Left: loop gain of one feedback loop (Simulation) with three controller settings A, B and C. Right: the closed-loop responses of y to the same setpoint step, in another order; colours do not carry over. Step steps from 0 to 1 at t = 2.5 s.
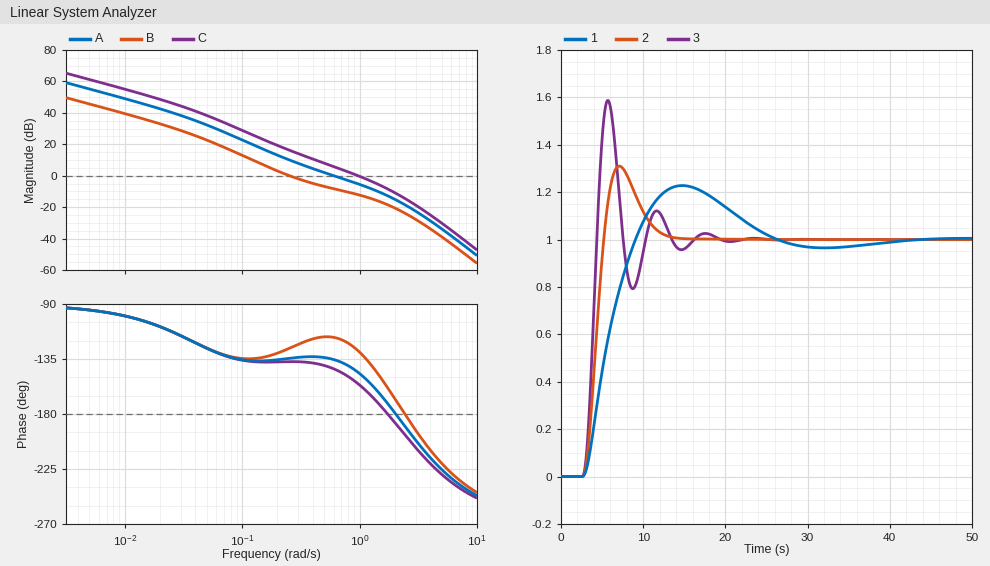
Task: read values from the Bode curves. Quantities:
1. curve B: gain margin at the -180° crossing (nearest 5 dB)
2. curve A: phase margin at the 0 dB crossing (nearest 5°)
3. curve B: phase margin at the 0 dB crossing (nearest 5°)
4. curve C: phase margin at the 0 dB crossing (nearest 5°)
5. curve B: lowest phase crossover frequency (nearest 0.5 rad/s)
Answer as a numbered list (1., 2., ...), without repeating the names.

1. 25 dB
2. 45°
3. 55°
4. 25°
5. 2.5 rad/s
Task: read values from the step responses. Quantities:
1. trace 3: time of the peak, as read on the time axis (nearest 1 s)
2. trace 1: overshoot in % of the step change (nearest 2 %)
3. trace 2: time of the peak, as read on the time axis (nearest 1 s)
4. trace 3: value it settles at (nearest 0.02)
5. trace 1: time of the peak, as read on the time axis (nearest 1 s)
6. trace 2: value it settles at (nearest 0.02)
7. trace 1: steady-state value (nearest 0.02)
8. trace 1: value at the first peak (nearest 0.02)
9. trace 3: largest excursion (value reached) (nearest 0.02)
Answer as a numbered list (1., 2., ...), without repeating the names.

1. 6 s
2. 22 %
3. 7 s
4. 1.00
5. 15 s
6. 1.00
7. 1.00
8. 1.22
9. 1.58
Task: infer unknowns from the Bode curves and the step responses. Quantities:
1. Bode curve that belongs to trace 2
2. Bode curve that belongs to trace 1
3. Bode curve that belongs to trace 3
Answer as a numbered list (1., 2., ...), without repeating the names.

1. A
2. B
3. C
